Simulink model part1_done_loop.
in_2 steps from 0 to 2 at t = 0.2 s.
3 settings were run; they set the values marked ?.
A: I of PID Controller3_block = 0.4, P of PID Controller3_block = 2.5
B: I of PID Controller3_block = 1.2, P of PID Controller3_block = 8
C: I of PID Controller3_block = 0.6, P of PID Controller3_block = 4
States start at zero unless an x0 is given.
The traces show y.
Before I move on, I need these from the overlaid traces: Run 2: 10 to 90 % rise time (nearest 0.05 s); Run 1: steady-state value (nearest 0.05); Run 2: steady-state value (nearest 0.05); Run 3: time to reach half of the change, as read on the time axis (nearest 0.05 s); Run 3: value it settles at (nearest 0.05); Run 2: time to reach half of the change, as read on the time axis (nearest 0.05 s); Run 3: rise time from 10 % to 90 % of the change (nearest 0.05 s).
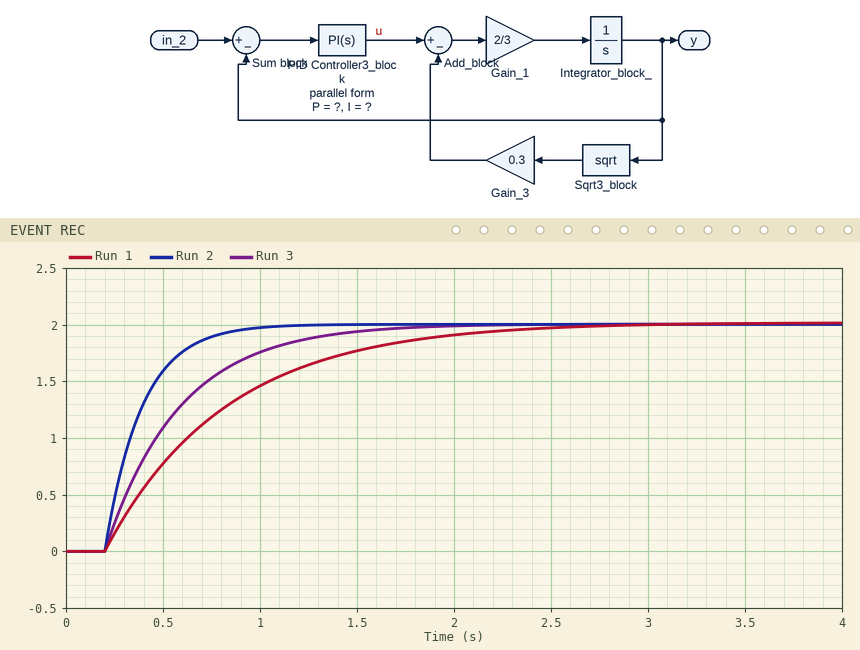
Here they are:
0.40 s
2.00
2.00
0.45 s
2.00
0.35 s
0.85 s
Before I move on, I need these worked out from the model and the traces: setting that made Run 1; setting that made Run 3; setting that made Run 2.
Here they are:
A
C
B
